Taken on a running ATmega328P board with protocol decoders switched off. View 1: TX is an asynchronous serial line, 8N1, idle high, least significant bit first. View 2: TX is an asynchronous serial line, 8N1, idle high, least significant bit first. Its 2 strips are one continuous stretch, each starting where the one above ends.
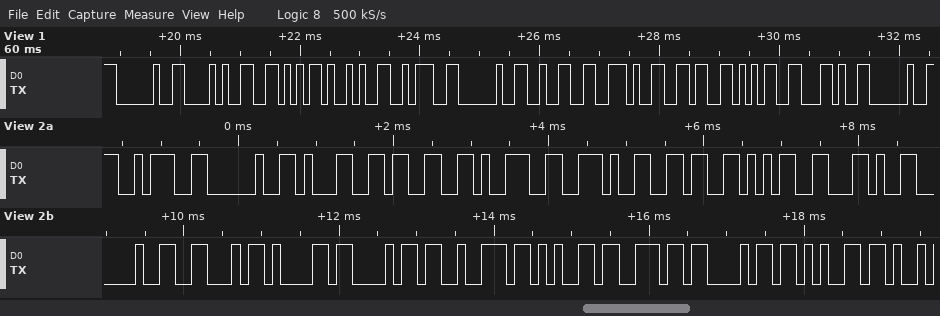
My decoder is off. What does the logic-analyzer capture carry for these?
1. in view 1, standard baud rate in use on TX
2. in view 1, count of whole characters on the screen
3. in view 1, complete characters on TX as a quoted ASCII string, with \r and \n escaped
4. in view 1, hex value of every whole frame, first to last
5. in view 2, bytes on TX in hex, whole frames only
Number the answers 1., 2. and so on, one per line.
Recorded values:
1. 9600 baud
2. 12
3. " (V): 2.65, "
4. 20 28 56 29 3A 20 32 2E 36 35 2C 20
5. 0x3A 0x20 0x31 0x33 0x39 0x2E 0x36 0x35 0x2C 0x20 0x46 0x61 0x68 0x72 0x65 0x6E 0x68 0x65
